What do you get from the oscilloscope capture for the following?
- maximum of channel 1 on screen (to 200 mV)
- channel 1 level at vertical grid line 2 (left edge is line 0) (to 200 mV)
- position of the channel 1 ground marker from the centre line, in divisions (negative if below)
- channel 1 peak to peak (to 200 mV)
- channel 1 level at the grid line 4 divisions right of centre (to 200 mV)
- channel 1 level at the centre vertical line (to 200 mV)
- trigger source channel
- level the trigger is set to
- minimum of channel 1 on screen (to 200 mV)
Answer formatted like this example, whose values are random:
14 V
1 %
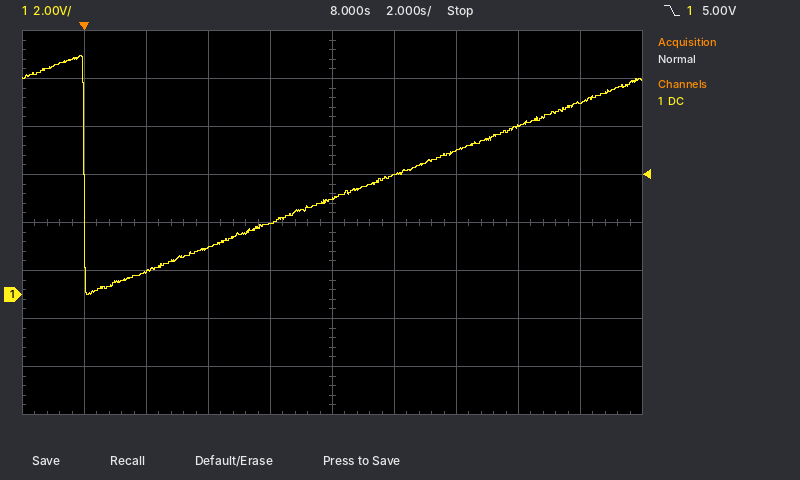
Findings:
10.0 V
1.0 V
-1.5 div
10.0 V
8.0 V
4.0 V
channel 1
5.00 V
0.0 V
